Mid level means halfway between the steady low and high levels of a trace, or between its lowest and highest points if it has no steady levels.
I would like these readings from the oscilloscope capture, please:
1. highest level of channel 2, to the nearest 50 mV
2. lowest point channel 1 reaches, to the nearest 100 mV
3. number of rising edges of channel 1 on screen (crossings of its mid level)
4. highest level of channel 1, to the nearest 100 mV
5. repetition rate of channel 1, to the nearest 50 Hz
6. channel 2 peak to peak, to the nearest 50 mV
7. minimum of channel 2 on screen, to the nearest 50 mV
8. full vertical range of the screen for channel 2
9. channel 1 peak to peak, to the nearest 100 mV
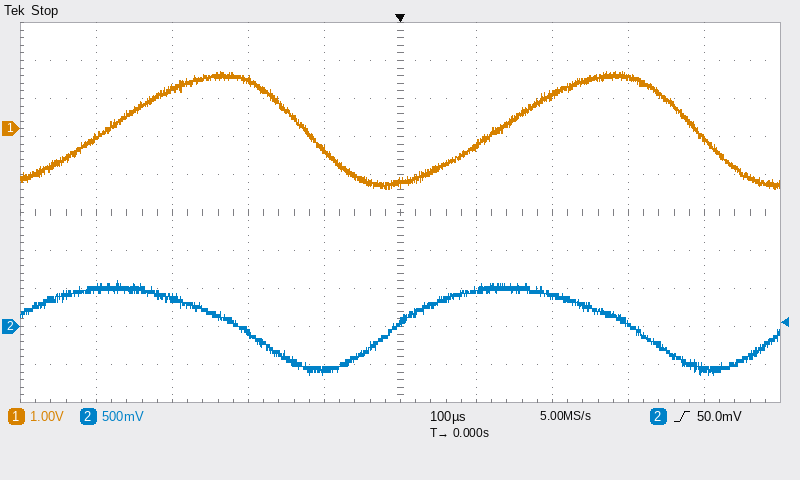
600 mV
-1.6 V
2
1.5 V
1.95 kHz
1.25 V
-650 mV
5 V
3.1 V
